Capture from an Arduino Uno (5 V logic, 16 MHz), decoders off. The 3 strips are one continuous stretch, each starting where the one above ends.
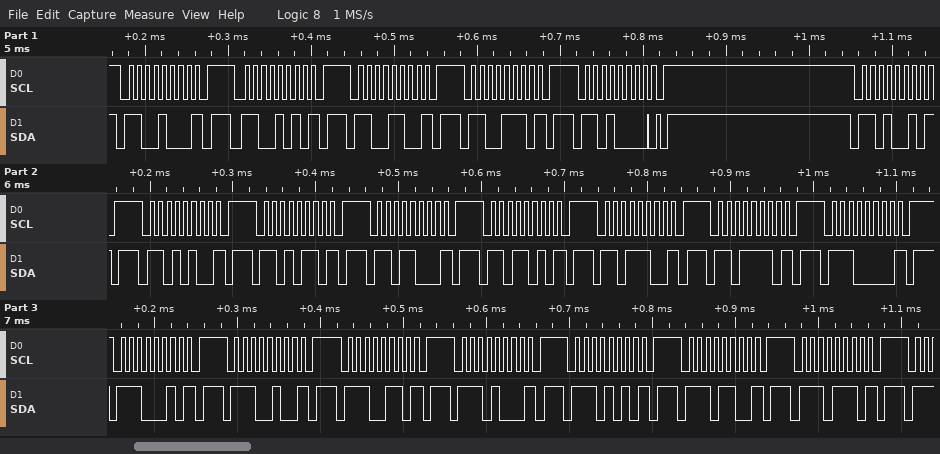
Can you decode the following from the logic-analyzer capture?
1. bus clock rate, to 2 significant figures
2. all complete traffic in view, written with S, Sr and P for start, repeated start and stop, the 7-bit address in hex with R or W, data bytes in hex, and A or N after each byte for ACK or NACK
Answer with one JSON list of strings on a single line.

["100 kHz", "S 64W N P S 65W N P S 66W N P S 67W N P S 68W A P S 69W N P S 6AW N P S 6BW N P S 6CW N P S 6DW N P S 6EW N P S 6FW N P S 70W N P S 71W N P S 72W N P S 73W N P S 74W N P S 75W N P S 76W N P S 77W N P"]
